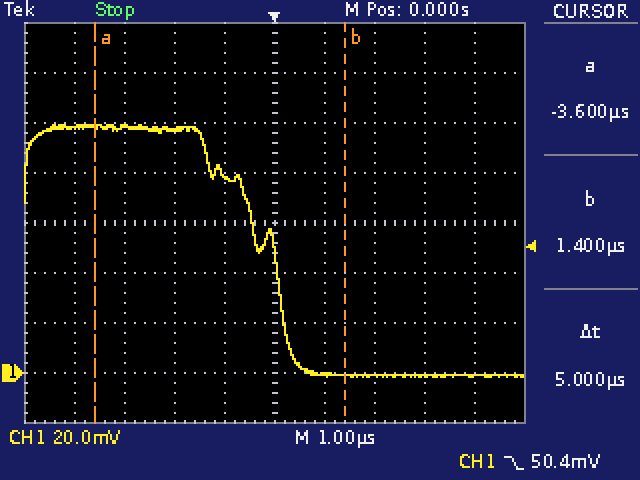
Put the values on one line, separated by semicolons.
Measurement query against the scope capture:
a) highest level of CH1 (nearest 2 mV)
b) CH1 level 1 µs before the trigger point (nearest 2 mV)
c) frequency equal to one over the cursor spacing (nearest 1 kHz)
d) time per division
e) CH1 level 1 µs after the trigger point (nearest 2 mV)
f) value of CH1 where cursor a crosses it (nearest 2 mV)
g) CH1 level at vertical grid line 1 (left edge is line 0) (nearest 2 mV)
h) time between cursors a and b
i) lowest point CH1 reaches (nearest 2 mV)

100 mV; 80 mV; 200 kHz; 1 µs; 0 mV; 98 mV; 98 mV; 5 µs; -2 mV
